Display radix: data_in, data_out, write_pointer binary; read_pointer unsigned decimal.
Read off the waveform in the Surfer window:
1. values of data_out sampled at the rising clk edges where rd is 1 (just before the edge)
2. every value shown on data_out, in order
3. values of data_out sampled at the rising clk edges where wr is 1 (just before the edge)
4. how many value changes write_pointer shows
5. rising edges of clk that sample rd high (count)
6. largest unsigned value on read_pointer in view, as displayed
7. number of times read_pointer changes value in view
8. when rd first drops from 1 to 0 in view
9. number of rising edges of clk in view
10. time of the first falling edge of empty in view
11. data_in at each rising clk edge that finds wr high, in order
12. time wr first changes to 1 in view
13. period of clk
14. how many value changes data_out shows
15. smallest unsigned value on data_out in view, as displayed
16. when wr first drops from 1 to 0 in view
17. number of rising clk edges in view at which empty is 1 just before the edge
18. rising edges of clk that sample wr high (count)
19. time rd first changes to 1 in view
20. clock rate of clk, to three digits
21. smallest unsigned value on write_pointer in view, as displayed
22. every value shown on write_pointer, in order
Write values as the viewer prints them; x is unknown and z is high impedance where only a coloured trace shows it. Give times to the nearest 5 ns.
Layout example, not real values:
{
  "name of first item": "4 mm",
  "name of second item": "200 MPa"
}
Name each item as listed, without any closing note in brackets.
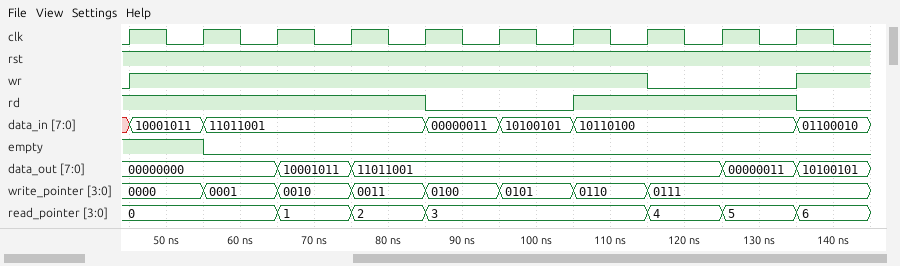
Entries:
{
  "values of data_out sampled at the rising clk edges where rd is 1": "00000000, 00000000, 00000000, 10001011, 11011001, 11011001, 11011001, 00000011",
  "every value shown on data_out, in order": "00000000, 10001011, 11011001, 00000011, 10100101",
  "values of data_out sampled at the rising clk edges where wr is 1": "00000000, 00000000, 10001011, 11011001, 11011001, 11011001, 11011001",
  "how many value changes write_pointer shows": "7",
  "rising edges of clk that sample rd high": "8",
  "largest unsigned value on read_pointer in view, as displayed": "6",
  "number of times read_pointer changes value in view": "6",
  "when rd first drops from 1 to 0 in view": "85 ns",
  "number of rising edges of clk in view": "10",
  "time of the first falling edge of empty in view": "55 ns",
  "data_in at each rising clk edge that finds wr high, in order": "10001011, 11011001, 11011001, 11011001, 00000011, 10100101, 10110100",
  "time wr first changes to 1 in view": "45 ns",
  "period of clk": "10 ns",
  "how many value changes data_out shows": "4",
  "smallest unsigned value on data_out in view, as displayed": "00000000",
  "when wr first drops from 1 to 0 in view": "115 ns",
  "number of rising clk edges in view at which empty is 1 just before the edge": "2",
  "rising edges of clk that sample wr high": "7",
  "time rd first changes to 1 in view": "105 ns",
  "clock rate of clk, to three digits": "100 MHz",
  "smallest unsigned value on write_pointer in view, as displayed": "0000",
  "every value shown on write_pointer, in order": "0000, 0001, 0010, 0011, 0100, 0101, 0110, 0111"
}
